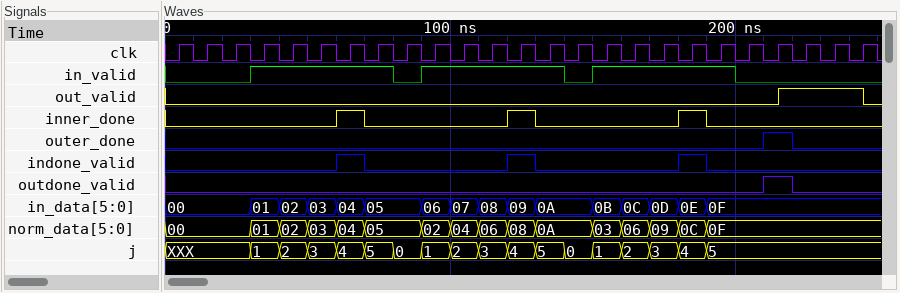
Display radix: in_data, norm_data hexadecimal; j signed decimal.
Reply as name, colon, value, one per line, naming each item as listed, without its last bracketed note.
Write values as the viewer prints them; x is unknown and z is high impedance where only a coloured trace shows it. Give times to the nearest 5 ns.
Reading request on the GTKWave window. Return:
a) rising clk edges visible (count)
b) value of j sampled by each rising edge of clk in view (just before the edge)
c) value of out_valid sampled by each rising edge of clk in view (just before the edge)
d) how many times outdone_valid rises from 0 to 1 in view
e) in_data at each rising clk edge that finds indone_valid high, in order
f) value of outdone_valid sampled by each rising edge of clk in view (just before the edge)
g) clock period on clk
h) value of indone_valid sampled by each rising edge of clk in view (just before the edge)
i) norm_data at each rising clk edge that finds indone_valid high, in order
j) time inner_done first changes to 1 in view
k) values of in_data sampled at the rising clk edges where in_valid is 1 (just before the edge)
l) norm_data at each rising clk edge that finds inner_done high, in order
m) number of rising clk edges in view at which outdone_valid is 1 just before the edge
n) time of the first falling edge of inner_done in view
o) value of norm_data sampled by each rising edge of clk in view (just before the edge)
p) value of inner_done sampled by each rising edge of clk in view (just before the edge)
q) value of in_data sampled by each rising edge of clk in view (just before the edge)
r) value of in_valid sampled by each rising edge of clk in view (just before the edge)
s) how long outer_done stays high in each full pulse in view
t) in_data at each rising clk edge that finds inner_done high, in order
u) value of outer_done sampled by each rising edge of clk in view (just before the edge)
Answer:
rising clk edges visible: 25
value of j sampled by each rising edge of clk in view: XXX, XXX, XXX, 1, 2, 3, 4, 5, 0, 1, 2, 3, 4, 5, 0, 1, 2, 3, 4, 5, 5, 5, 5, 5, 5
value of out_valid sampled by each rising edge of clk in view: 0 0 0 0 0 0 0 0 0 0 0 0 0 0 0 0 0 0 0 0 0 0 1 1 1
how many times outdone_valid rises from 0 to 1 in view: 1
in_data at each rising clk edge that finds indone_valid high, in order: 04, 09, 0E
value of outdone_valid sampled by each rising edge of clk in view: 0 0 0 0 0 0 0 0 0 0 0 0 0 0 0 0 0 0 0 0 0 1 0 0 0
clock period on clk: 10 ns
value of indone_valid sampled by each rising edge of clk in view: 0 0 0 0 0 0 1 0 0 0 0 0 1 0 0 0 0 0 1 0 0 0 0 0 0
norm_data at each rising clk edge that finds indone_valid high, in order: 04, 08, 0C
time inner_done first changes to 1 in view: 60 ns
values of in_data sampled at the rising clk edges where in_valid is 1: 01, 02, 03, 04, 05, 06, 07, 08, 09, 0A, 0B, 0C, 0D, 0E, 0F
norm_data at each rising clk edge that finds inner_done high, in order: 04, 08, 0C
number of rising clk edges in view at which outdone_valid is 1 just before the edge: 1
time of the first falling edge of inner_done in view: 70 ns
value of norm_data sampled by each rising edge of clk in view: 00, 00, 00, 01, 02, 03, 04, 05, 05, 02, 04, 06, 08, 0A, 0A, 03, 06, 09, 0C, 0F, 0F, 0F, 0F, 0F, 0F
value of inner_done sampled by each rising edge of clk in view: 0 0 0 0 0 0 1 0 0 0 0 0 1 0 0 0 0 0 1 0 0 0 0 0 0
value of in_data sampled by each rising edge of clk in view: 00, 00, 00, 01, 02, 03, 04, 05, 05, 06, 07, 08, 09, 0A, 0A, 0B, 0C, 0D, 0E, 0F, 0F, 0F, 0F, 0F, 0F
value of in_valid sampled by each rising edge of clk in view: 0 0 0 1 1 1 1 1 0 1 1 1 1 1 0 1 1 1 1 1 0 0 0 0 0
how long outer_done stays high in each full pulse in view: 10 ns
in_data at each rising clk edge that finds inner_done high, in order: 04, 09, 0E
value of outer_done sampled by each rising edge of clk in view: 0 0 0 0 0 0 0 0 0 0 0 0 0 0 0 0 0 0 0 0 0 1 0 0 0
